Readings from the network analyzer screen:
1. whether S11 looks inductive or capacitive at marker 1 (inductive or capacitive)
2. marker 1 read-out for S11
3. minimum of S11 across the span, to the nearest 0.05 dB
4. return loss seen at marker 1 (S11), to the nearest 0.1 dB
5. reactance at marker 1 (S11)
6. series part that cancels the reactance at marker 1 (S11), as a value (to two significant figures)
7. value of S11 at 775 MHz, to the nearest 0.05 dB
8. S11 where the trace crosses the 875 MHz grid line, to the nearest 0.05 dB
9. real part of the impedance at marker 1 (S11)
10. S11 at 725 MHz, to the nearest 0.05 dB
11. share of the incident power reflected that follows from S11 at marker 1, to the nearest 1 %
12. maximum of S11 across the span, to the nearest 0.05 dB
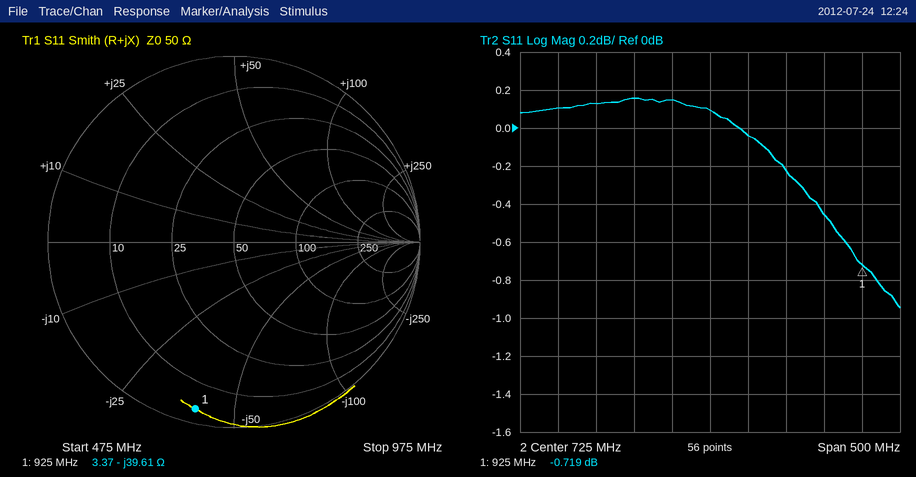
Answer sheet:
capacitive
-0.719 dB
-0.95 dB
0.7 dB
-39.61 Ω
6.8 nH
-0.05 dB
-0.45 dB
3.37 Ω
0.10 dB
85 %
0.15 dB
